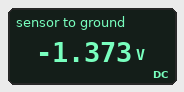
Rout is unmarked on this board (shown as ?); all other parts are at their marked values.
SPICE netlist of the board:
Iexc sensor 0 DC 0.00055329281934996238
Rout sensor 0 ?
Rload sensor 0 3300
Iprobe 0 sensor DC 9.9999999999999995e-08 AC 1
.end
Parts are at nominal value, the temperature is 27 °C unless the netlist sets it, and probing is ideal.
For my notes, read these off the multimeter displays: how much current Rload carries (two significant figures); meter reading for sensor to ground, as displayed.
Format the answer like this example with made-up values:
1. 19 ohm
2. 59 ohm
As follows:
1. 420 µA
2. -1.373 V
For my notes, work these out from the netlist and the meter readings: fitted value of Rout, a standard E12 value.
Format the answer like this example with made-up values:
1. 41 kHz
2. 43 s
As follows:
1. 10 kΩ
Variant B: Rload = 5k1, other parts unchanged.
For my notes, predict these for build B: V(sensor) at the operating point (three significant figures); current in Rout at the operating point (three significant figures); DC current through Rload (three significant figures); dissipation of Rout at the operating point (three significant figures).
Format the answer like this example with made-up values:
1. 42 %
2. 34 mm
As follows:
1. -1.87 V
2. 187 µA
3. 366 µA
4. 349 µW
